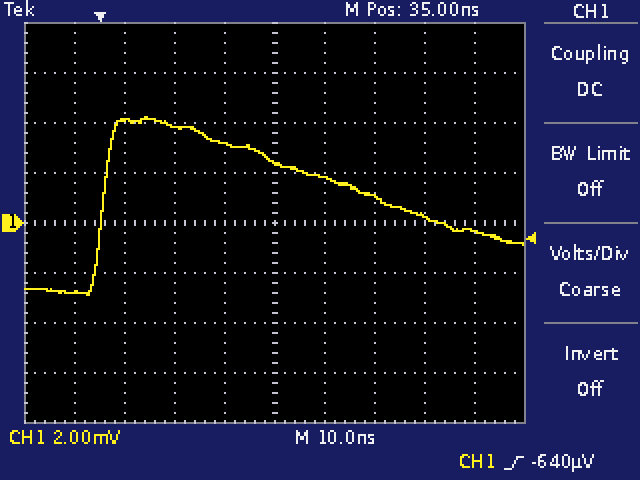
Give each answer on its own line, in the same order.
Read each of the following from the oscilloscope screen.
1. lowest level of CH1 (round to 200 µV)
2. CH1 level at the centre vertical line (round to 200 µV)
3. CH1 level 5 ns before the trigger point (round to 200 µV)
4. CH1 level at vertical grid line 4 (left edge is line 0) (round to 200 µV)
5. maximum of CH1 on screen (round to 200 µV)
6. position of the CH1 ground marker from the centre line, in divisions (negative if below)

-2.8 mV
2.4 mV
-2.8 mV
3.2 mV
4.2 mV
0.0 div
